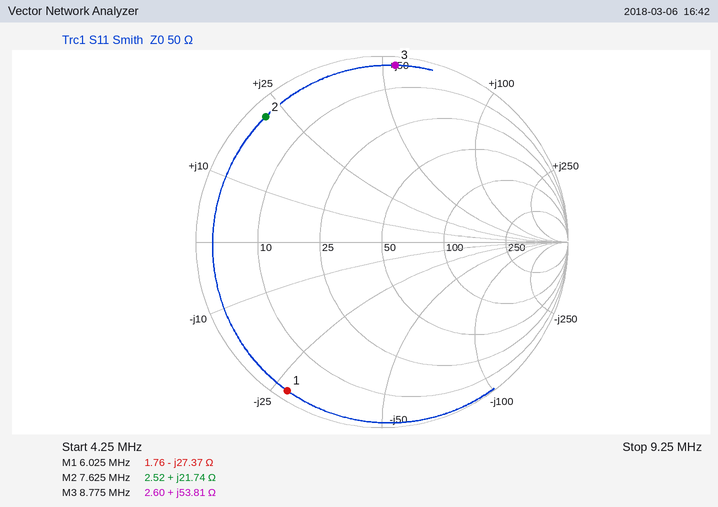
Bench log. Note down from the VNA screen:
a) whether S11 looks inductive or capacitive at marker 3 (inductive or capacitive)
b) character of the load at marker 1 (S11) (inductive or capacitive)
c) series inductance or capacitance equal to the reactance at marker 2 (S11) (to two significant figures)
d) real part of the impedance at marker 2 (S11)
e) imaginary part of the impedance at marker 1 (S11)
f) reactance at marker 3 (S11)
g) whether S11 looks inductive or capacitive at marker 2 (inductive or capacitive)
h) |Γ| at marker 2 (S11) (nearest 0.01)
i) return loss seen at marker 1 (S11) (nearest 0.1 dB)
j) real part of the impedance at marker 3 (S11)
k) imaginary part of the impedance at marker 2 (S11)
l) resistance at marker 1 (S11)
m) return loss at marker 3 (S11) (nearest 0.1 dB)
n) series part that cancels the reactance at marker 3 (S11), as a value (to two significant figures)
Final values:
inductive
capacitive
450 nH
2.52 Ω
-27.37 Ω
+53.81 Ω
inductive
0.92
0.5 dB
2.60 Ω
+21.74 Ω
1.76 Ω
0.4 dB
340 pF
